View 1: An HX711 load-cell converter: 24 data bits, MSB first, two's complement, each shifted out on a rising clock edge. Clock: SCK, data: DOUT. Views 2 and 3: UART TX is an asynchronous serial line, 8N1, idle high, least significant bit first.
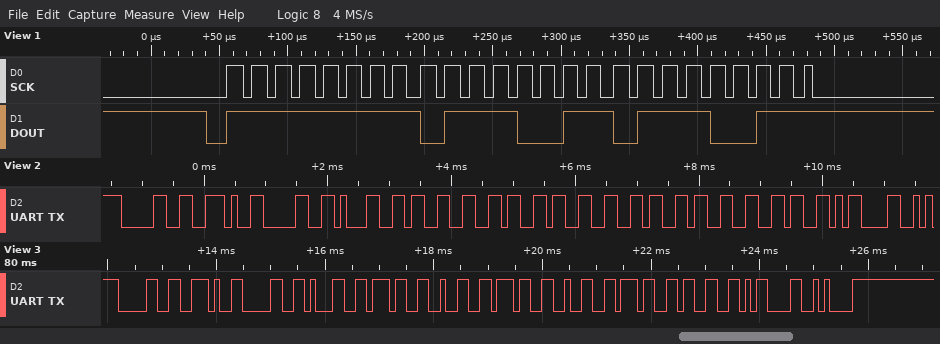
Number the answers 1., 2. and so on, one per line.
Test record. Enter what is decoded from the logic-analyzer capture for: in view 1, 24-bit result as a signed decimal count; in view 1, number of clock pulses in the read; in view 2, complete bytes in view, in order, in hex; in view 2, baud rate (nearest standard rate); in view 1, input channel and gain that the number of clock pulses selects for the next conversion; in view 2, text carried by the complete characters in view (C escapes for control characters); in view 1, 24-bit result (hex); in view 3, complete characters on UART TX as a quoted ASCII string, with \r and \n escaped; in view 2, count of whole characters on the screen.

1. -35981
2. 25
3. 30 2E 30 31 33 36 33 36 33 36 0D
4. 9600 baud
5. channel A, gain 128
6. "0.01363636\r"
7. 0xFF7373
8. "0.01727273\r\n"
9. 11
